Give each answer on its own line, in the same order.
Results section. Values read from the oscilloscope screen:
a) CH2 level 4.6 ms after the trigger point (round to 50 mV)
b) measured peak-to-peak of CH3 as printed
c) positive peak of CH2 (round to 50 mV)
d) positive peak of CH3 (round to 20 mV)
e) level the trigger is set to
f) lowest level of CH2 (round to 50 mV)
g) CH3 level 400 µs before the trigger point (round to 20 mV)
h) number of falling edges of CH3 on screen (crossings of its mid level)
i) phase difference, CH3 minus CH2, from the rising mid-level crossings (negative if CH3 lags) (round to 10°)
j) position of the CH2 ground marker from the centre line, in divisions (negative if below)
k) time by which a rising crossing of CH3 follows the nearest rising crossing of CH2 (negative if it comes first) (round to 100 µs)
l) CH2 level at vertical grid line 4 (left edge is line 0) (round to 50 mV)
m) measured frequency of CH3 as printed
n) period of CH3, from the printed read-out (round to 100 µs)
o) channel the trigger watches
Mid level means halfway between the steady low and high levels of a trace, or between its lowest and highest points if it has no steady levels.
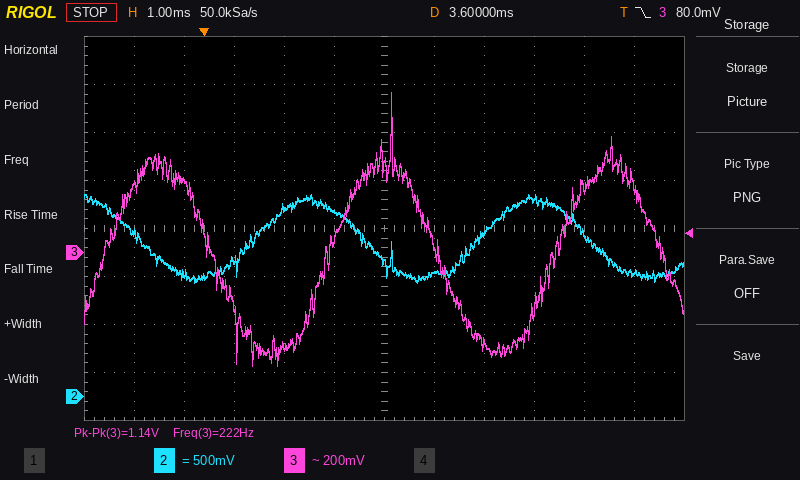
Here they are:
1.30 V
1.14 V
2.10 V
660 mV
80.0 mV
1.20 V
300 mV
3
-140°
-3.5 div
+1.7 ms
1.95 V
222 Hz
4.5 ms
CH3
